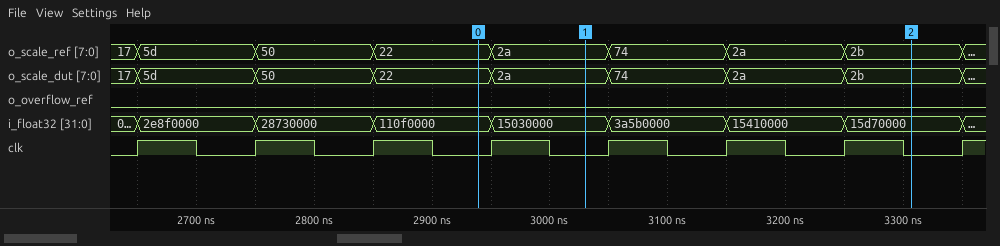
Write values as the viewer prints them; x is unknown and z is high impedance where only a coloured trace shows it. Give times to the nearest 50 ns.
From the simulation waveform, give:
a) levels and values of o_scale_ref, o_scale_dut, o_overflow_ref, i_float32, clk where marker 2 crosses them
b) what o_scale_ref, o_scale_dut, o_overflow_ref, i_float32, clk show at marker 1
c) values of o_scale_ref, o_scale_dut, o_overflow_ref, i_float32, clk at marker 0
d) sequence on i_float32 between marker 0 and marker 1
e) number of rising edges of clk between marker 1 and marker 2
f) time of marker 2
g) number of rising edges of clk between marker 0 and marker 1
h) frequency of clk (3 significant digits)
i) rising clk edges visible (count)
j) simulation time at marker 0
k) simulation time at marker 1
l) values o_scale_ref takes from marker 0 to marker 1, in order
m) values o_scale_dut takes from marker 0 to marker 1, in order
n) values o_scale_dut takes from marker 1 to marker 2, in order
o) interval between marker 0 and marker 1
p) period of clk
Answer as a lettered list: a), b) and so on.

a) o_scale_ref=2b, o_scale_dut=2b, o_overflow_ref=0, i_float32=15d70000, clk=0
b) o_scale_ref=2a, o_scale_dut=2a, o_overflow_ref=0, i_float32=15030000, clk=0
c) o_scale_ref=22, o_scale_dut=22, o_overflow_ref=0, i_float32=110f0000, clk=0
d) 110f0000, 15030000
e) 3
f) 3300 ns
g) 1
h) 10.0 MHz
i) 8
j) 2950 ns
k) 3050 ns
l) 22, 2a
m) 22, 2a
n) 2a, 74, 2a, 2b
o) 100 ns
p) 100 ns
